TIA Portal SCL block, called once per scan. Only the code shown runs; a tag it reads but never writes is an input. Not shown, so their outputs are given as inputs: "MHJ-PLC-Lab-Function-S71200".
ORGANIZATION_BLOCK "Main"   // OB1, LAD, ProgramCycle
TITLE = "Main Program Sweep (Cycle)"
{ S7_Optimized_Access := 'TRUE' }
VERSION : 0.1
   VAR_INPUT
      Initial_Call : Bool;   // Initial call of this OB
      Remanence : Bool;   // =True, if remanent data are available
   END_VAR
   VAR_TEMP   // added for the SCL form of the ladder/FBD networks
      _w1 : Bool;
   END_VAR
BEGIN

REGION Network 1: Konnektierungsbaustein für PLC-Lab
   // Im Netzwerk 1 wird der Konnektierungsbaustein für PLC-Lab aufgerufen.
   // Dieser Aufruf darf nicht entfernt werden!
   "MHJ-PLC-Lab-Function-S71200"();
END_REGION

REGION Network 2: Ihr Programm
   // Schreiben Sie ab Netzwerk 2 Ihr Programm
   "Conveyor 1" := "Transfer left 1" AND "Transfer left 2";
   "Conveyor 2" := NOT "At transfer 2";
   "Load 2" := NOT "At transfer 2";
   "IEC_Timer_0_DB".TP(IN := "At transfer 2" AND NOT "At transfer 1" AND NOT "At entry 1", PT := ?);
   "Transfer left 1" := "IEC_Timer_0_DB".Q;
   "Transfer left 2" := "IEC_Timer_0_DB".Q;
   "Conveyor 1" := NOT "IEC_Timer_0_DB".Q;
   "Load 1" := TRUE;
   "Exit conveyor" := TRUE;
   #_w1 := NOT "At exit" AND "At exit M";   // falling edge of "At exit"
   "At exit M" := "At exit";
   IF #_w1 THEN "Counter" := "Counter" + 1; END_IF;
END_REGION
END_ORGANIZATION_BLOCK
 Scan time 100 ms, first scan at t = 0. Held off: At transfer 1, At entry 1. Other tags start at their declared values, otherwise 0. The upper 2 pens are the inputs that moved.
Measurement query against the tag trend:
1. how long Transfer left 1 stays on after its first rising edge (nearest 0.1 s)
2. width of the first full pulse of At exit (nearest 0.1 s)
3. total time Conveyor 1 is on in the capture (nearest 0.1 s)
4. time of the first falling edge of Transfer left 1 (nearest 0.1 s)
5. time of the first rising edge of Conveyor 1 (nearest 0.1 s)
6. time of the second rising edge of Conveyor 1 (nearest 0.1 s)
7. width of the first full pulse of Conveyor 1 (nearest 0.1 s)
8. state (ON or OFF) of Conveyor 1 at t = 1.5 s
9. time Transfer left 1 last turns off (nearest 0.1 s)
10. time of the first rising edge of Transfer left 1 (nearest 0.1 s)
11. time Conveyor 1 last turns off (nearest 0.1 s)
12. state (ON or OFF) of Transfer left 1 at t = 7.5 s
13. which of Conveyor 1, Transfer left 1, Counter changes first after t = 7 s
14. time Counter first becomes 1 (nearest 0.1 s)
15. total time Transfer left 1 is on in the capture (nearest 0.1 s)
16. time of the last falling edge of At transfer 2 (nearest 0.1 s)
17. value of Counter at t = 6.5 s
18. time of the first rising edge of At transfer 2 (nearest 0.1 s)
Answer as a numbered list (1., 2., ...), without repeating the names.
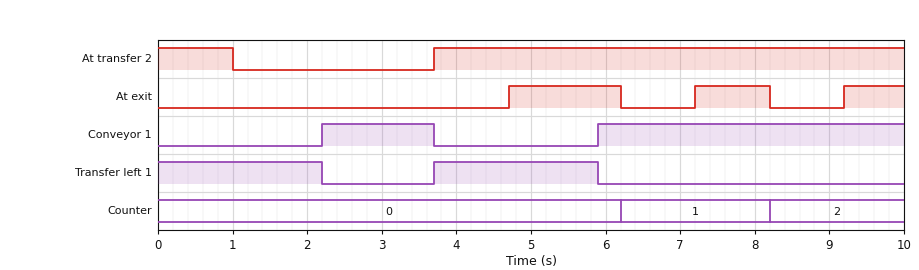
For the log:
1. 2.2 s
2. 1.5 s
3. 5.6 s
4. 2.2 s
5. 2.2 s
6. 5.9 s
7. 1.5 s
8. OFF
9. 5.9 s
10. 3.7 s
11. 3.7 s
12. OFF
13. Counter
14. 6.2 s
15. 4.4 s
16. 1.0 s
17. 1
18. 3.7 s
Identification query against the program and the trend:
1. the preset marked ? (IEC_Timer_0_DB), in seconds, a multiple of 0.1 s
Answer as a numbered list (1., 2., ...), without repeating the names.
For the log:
1. 2.2 s
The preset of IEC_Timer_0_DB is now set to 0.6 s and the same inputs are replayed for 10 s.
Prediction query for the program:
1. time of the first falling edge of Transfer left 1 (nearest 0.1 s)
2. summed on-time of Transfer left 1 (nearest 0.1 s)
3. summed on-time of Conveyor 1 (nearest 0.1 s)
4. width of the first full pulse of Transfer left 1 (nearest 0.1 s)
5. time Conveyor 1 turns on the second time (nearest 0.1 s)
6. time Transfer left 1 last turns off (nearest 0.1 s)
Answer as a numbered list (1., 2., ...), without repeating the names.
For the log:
1. 0.6 s
2. 1.2 s
3. 8.8 s
4. 0.6 s
5. 4.3 s
6. 4.3 s
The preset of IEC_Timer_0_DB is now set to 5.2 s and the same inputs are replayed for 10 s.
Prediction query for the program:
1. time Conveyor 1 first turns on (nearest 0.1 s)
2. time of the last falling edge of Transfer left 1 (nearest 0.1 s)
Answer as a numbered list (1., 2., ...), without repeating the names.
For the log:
1. 5.2 s
2. 5.2 s
